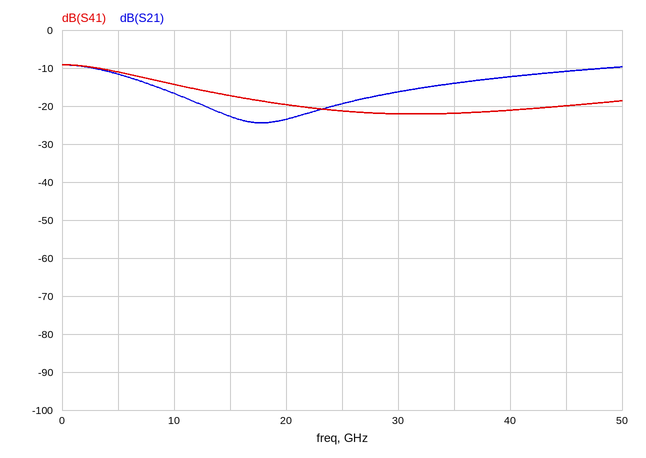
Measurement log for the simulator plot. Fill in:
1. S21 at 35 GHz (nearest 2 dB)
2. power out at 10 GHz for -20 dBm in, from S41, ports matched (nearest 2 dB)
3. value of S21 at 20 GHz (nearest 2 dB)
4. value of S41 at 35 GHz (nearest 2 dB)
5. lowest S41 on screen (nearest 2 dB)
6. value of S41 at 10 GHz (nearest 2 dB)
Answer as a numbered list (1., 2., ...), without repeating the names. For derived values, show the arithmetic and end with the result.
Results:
1. -14 dB
2. -20 dBm + (-14 dB) = -34 dBm
3. -24 dB
4. -22 dB
5. -22 dB
6. -14 dB
